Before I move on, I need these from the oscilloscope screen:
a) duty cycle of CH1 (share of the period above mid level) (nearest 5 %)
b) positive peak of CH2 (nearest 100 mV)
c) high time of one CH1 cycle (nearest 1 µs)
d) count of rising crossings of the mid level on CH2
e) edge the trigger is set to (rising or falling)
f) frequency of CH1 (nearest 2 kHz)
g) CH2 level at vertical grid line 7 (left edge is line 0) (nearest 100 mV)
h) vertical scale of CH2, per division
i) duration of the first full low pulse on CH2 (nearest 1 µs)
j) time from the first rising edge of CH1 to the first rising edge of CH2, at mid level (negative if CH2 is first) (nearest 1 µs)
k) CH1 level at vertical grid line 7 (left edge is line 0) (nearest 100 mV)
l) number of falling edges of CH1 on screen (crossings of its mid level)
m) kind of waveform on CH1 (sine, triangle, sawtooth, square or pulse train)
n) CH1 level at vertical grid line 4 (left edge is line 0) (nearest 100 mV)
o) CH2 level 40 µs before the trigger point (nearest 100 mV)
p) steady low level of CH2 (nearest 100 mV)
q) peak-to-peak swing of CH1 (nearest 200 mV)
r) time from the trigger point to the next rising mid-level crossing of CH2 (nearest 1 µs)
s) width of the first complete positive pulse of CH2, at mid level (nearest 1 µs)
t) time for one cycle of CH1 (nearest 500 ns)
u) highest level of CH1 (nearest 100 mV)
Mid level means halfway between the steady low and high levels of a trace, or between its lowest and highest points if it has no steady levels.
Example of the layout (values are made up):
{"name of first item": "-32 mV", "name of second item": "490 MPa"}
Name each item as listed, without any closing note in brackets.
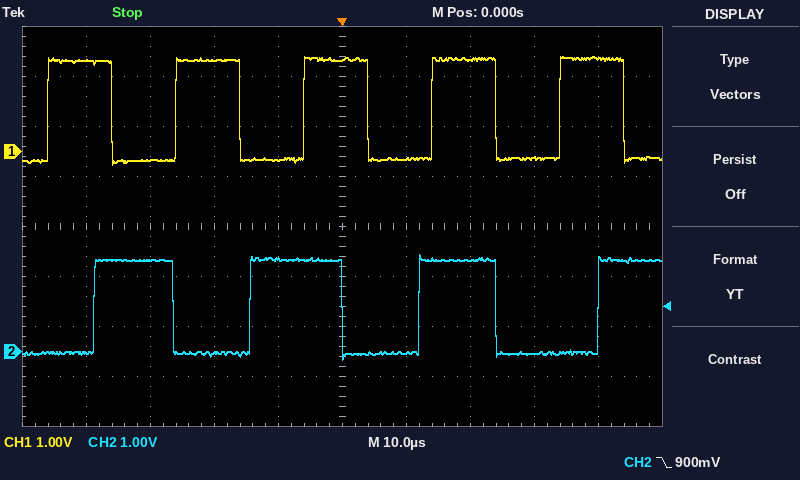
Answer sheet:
{"duty cycle of CH1 (share of the period above mid level)": "50 %", "positive peak of CH2": "1.9 V", "high time of one CH1 cycle": "10 µs", "count of rising crossings of the mid level on CH2": "4", "edge the trigger is set to": "falling", "frequency of CH1": "50 kHz", "CH2 level at vertical grid line 7 (left edge is line 0)": "1.8 V", "vertical scale of CH2, per division": "1 V", "duration of the first full low pulse on CH2": "12 µs", "time from the first rising edge of CH1 to the first rising edge of CH2, at mid level (negative if CH2 is first)": "+7 µs", "CH1 level at vertical grid line 7 (left edge is line 0)": "1.8 V", "number of falling edges of CH1 on screen": "5", "kind of waveform on CH1": "square", "CH1 level at vertical grid line 4 (left edge is line 0)": "-200 mV", "CH2 level 40 µs before the trigger point": "0.0 V", "steady low level of CH2": "0.0 V", "peak-to-peak swing of CH1": "2.2 V", "time from the trigger point to the next rising mid-level crossing of CH2": "12 µs", "width of the first complete positive pulse of CH2, at mid level": "12 µs", "time for one cycle of CH1": "20.0 µs", "highest level of CH1": "1.9 V"}
